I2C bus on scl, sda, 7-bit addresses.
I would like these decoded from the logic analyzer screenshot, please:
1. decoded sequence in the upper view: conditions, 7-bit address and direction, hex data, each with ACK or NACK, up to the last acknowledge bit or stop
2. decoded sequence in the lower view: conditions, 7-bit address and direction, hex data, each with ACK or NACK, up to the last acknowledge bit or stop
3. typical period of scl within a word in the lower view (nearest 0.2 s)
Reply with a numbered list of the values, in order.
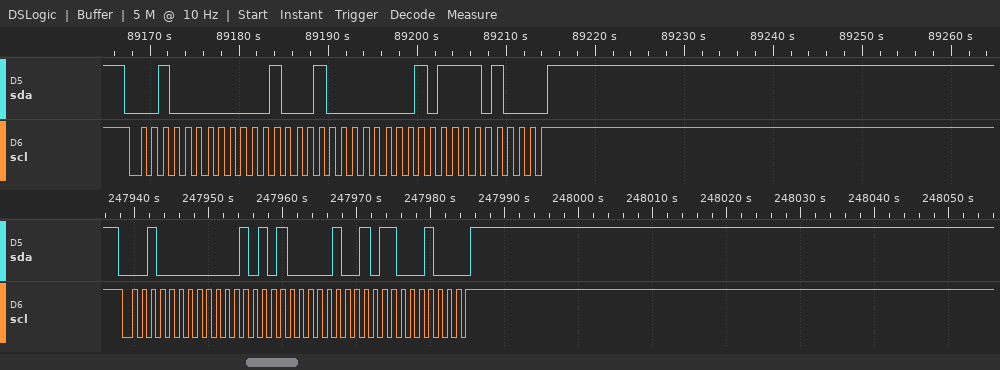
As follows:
1. start, address 10 write ACK, 11 ACK, 01 ACK, F4 ACK, stop
2. start, address 10 write ACK, 15 ACK, 09 ACK, C4 ACK, stop
3. 1.2 s
